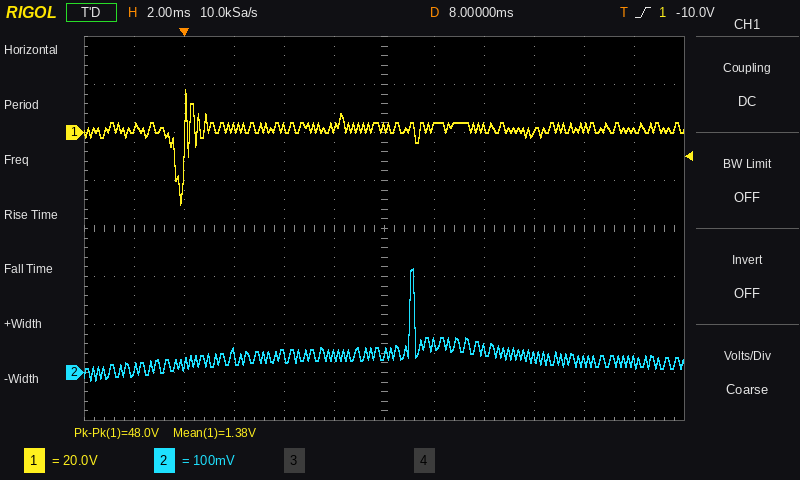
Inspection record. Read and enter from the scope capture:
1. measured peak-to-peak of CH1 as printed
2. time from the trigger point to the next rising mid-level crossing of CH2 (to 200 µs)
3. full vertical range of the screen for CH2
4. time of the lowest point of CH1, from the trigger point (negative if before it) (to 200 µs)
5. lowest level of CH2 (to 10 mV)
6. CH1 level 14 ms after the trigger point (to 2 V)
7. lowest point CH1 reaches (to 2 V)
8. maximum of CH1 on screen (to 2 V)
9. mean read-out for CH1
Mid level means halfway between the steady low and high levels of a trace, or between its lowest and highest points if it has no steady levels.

48.0 V
9.0 ms
800 mV
-200 µs
-20 mV
0 V
-30 V
18 V
1.38 V
